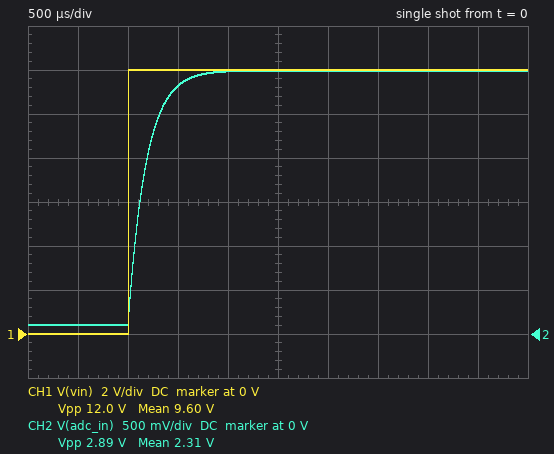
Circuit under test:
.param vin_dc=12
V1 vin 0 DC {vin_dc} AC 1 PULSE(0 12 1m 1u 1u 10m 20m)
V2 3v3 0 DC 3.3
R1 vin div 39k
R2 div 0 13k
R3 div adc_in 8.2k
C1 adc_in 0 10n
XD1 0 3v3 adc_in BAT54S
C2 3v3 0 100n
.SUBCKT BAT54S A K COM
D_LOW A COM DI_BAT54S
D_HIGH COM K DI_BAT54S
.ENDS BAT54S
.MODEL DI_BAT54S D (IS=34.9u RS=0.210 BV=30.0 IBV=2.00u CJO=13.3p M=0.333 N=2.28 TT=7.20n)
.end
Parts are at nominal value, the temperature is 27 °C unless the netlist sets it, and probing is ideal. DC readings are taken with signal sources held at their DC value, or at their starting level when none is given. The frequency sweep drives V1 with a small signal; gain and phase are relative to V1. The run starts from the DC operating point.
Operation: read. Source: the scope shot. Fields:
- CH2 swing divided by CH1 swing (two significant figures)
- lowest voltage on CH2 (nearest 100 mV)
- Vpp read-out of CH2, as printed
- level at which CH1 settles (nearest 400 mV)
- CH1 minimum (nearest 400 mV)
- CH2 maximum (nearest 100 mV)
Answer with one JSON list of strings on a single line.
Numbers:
["0.24", "100 mV", "2.89 V", "12.0 V", "0 V", "3.0 V"]
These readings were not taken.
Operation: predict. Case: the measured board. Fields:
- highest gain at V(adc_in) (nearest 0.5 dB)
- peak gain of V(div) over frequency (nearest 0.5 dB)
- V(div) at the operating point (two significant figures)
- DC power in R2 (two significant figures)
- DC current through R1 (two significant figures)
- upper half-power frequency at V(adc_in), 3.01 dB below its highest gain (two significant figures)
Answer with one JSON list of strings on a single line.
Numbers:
["-12.5 dB", "-12.5 dB", "3.0 V", "690 µW", "230 µA", "940 Hz"]
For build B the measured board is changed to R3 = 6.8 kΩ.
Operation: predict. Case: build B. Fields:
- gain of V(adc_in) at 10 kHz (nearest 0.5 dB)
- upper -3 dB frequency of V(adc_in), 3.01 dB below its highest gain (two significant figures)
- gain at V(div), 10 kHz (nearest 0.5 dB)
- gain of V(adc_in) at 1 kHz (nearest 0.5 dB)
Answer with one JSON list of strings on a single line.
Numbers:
["-32.5 dB", "1.0 kHz", "-19.5 dB", "-15.5 dB"]
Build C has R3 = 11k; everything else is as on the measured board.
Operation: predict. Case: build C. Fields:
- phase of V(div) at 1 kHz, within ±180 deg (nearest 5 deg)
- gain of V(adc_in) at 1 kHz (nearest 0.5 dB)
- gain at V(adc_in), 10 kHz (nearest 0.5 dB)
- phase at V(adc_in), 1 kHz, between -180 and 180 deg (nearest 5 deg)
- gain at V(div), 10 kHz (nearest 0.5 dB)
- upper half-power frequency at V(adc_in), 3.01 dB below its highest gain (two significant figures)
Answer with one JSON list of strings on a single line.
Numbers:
["-15 deg", "-16.5 dB", "-34.5 dB", "-50 deg", "-17.5 dB", "820 Hz"]
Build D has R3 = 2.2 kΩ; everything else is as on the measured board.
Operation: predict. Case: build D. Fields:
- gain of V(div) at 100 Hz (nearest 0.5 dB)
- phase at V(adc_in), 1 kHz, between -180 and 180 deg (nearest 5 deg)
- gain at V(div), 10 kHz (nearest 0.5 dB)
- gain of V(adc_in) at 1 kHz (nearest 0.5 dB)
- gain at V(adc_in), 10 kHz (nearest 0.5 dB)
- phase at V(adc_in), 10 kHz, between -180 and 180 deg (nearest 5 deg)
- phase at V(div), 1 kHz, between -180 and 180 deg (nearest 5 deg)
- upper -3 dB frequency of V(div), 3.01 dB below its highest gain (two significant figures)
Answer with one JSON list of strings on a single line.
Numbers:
["-12.5 dB", "-35 deg", "-25.0 dB", "-14.0 dB", "-29.5 dB", "-80 deg", "-30 deg", "1.4 kHz"]
